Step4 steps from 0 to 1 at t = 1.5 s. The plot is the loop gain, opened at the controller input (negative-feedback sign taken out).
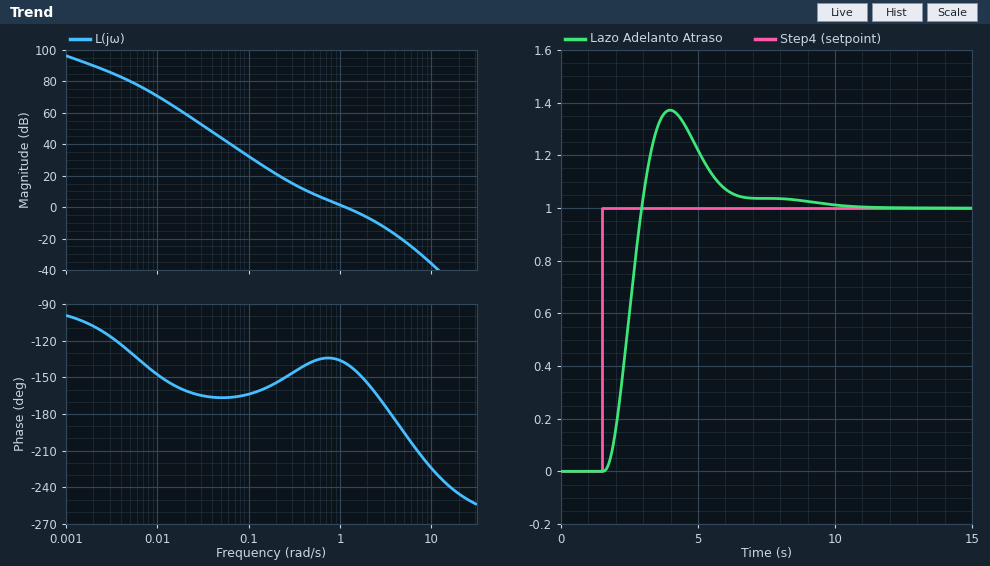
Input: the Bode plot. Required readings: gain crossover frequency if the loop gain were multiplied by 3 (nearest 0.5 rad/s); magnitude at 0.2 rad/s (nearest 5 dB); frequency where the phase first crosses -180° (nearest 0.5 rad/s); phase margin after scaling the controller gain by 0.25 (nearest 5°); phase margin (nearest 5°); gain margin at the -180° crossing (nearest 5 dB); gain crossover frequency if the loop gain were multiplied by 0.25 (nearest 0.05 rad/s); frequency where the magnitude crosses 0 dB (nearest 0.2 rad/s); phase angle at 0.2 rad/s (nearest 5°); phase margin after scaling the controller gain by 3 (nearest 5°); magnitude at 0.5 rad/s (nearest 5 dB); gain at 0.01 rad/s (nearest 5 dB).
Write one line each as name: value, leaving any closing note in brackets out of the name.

gain crossover frequency if the loop gain were multiplied by 3: 2.5 rad/s
magnitude at 0.2 rad/s: 20 dB
frequency where the phase first crosses -180°: 3.5 rad/s
phase margin after scaling the controller gain by 0.25: 40°
phase margin: 40°
gain margin at the -180° crossing: 15 dB
gain crossover frequency if the loop gain were multiplied by 0.25: 0.40 rad/s
frequency where the magnitude crosses 0 dB: 1.2 rad/s
phase angle at 0.2 rad/s: -155°
phase margin after scaling the controller gain by 3: 15°
magnitude at 0.5 rad/s: 10 dB
gain at 0.01 rad/s: 70 dB
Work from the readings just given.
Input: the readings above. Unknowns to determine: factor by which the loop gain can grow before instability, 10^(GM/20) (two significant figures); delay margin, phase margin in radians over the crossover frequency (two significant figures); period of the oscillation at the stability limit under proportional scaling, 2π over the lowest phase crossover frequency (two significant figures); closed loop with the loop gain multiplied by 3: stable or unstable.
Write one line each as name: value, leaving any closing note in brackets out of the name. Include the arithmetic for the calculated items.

factor by which the loop gain can grow before instability, 10^(GM/20): 10^(15 / 20) = 5.6
delay margin, phase margin in radians over the crossover frequency: 40 × π / 180 / 1.2 = 0.58 s
period of the oscillation at the stability limit under proportional scaling, 2π over the lowest phase crossover frequency: 2π / 3.5 = 1.8 s
closed loop with the loop gain multiplied by 3: stable or unstable: stable
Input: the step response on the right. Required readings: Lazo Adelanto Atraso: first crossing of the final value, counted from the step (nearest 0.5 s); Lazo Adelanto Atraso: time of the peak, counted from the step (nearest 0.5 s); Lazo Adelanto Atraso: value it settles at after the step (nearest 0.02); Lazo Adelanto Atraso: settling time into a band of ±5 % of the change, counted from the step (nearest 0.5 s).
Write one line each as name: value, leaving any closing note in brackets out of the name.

Lazo Adelanto Atraso: first crossing of the final value, counted from the step: 1.5 s
Lazo Adelanto Atraso: time of the peak, counted from the step: 2.5 s
Lazo Adelanto Atraso: value it settles at after the step: 1.00
Lazo Adelanto Atraso: settling time into a band of ±5 % of the change, counted from the step: 5.0 s
